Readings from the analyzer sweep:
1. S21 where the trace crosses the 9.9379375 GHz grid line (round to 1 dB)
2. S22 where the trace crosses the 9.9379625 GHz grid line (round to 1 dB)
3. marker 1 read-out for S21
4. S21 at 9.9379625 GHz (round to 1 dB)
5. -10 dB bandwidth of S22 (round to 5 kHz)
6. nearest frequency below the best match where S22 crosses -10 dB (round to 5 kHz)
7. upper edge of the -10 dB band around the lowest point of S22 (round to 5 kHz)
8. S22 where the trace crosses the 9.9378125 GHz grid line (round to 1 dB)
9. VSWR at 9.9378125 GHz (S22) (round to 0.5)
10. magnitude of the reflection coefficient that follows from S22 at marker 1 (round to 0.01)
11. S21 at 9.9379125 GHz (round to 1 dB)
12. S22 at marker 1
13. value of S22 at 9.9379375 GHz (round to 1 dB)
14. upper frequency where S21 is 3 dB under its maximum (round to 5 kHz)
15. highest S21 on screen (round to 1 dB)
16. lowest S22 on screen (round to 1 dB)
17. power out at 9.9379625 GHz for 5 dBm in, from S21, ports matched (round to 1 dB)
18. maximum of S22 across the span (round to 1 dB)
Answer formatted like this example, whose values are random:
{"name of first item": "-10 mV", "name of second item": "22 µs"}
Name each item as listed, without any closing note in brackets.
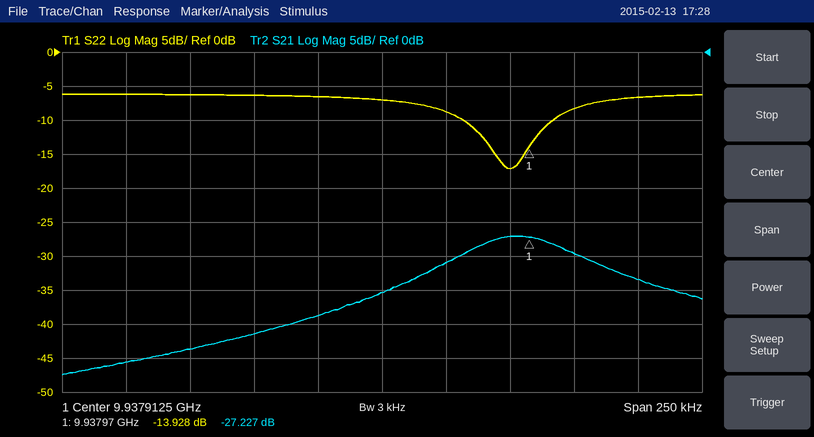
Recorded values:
{"S21 where the trace crosses the 9.9379375 GHz grid line": "-31 dB", "S22 where the trace crosses the 9.9379625 GHz grid line": "-17 dB", "marker 1 read-out for S21": "-27.227 dB", "S21 at 9.9379625 GHz": "-27 dB", "-10 dB bandwidth of S22": "35 kHz", "nearest frequency below the best match where S22 crosses -10 dB": "9.937945 GHz", "upper edge of the -10 dB band around the lowest point of S22": "9.937980 GHz", "S22 where the trace crosses the 9.9378125 GHz grid line": "-6 dB", "VSWR at 9.9378125 GHz (S22)": "3.0", "magnitude of the reflection coefficient that follows from S22 at marker 1": "0.20", "S21 at 9.9379125 GHz": "-35 dB", "S22 at marker 1": "-13.928 dB", "value of S22 at 9.9379375 GHz": "-9 dB", "upper frequency where S21 is 3 dB under its maximum": "9.937990 GHz", "highest S21 on screen": "-27 dB", "lowest S22 on screen": "-17 dB", "power out at 9.9379625 GHz for 5 dBm in, from S21, ports matched": "-22 dBm", "maximum of S22 across the span": "-6 dB"}
